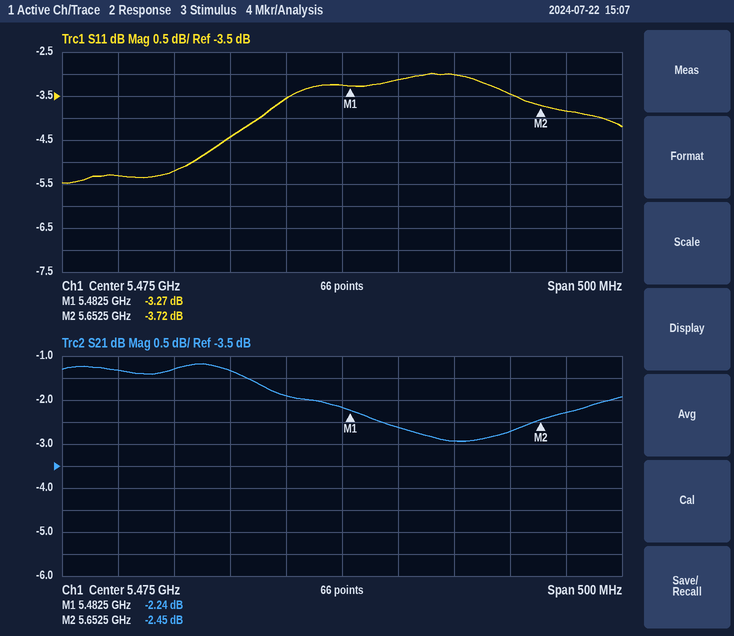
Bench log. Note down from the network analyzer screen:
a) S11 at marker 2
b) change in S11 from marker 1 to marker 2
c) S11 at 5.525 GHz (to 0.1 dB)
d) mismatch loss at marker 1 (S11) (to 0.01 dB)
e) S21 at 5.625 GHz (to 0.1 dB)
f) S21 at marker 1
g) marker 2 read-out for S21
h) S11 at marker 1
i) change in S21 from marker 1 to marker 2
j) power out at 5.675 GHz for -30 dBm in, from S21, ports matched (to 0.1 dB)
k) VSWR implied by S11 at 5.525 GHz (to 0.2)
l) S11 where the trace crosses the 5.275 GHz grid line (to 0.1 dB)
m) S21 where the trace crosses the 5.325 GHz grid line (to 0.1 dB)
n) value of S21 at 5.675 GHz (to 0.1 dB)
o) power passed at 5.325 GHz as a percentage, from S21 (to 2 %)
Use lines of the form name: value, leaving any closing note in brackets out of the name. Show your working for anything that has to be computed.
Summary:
S11 at marker 2: -3.72 dB
change in S11 from marker 1 to marker 2: -3.72 − (-3.27) = -0.45 dB
S11 at 5.525 GHz: -3.1 dB
mismatch loss at marker 1 (S11): −10 log10(1 − 10^(-3.27/10)) ≈ 2.77 dB
S21 at 5.625 GHz: -2.7 dB
S21 at marker 1: -2.24 dB
marker 2 read-out for S21: -2.45 dB
S11 at marker 1: -3.27 dB
change in S21 from marker 1 to marker 2: -2.45 − (-2.24) = -0.21 dB
power out at 5.675 GHz for -30 dBm in, from S21, ports matched: -30 dBm + (-2.3 dB) = -32.3 dBm
VSWR implied by S11 at 5.525 GHz: |Γ| = 10^(-3.1/20) = 0.6998; VSWR = (1 + 0.6998)/(1 − 0.6998) ≈ 5.66, so 5.6 to the nearest 0.2
S11 where the trace crosses the 5.275 GHz grid line: -5.3 dB
S21 where the trace crosses the 5.325 GHz grid line: -1.3 dB
value of S21 at 5.675 GHz: -2.3 dB
power passed at 5.325 GHz as a percentage, from S21: 10^(-1.3/10) ≈ 74 %
